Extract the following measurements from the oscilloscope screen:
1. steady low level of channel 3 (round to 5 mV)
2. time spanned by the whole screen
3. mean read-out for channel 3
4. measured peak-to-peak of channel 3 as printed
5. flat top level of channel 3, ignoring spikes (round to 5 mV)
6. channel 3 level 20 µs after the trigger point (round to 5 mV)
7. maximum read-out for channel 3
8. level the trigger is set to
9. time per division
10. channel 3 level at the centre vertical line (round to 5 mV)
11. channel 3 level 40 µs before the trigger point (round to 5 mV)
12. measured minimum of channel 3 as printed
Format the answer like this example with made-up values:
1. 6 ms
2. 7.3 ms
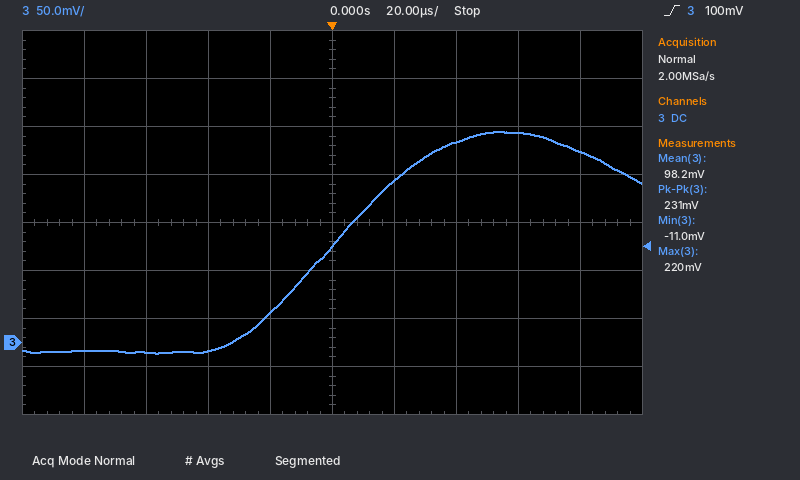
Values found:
1. -10 mV
2. 200 µs
3. 98.2 mV
4. 231 mV
5. 220 mV
6. 170 mV
7. 220 mV
8. 100 mV
9. 20 µs
10. 100 mV
11. -10 mV
12. -11.0 mV
